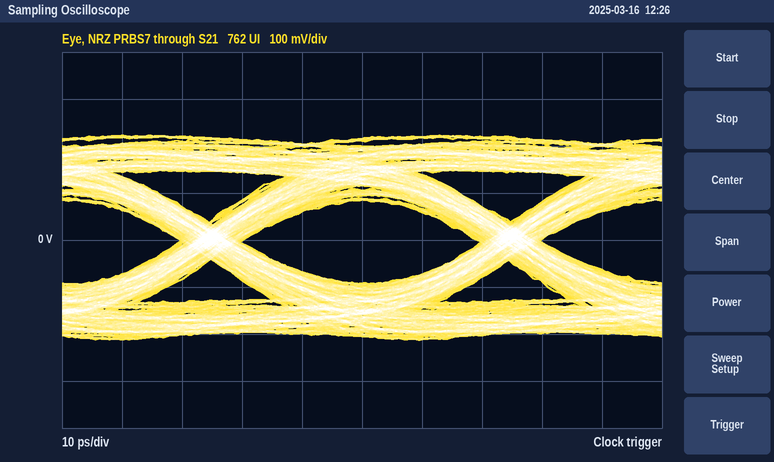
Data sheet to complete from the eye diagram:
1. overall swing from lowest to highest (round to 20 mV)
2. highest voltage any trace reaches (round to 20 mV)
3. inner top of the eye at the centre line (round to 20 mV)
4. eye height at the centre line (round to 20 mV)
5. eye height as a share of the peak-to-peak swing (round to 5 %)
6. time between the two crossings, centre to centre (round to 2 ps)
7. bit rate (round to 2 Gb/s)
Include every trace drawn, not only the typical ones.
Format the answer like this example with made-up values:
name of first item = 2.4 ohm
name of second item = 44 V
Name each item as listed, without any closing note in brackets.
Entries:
overall swing from lowest to highest = 440 mV
highest voltage any trace reaches = 220 mV
inner top of the eye at the centre line = 80 mV
eye height at the centre line = 180 mV
eye height as a share of the peak-to-peak swing = 40 %
time between the two crossings, centre to centre = 50 ps
bit rate = 20 Gb/s
